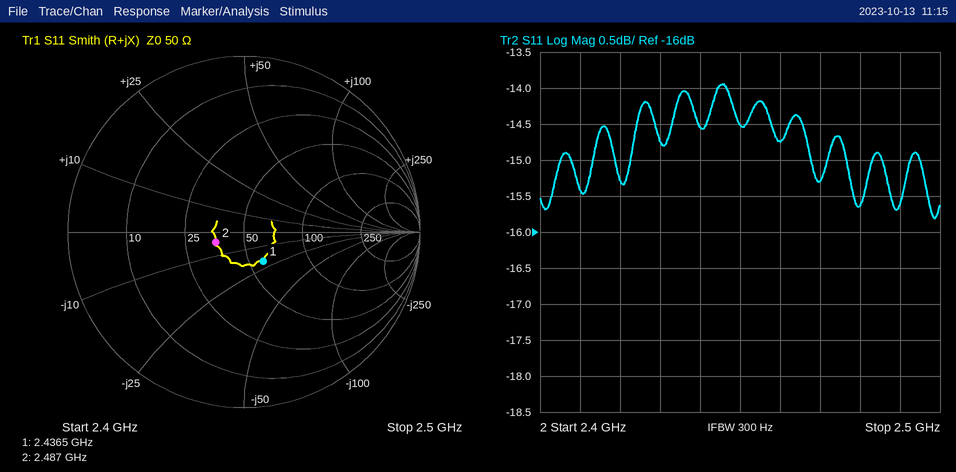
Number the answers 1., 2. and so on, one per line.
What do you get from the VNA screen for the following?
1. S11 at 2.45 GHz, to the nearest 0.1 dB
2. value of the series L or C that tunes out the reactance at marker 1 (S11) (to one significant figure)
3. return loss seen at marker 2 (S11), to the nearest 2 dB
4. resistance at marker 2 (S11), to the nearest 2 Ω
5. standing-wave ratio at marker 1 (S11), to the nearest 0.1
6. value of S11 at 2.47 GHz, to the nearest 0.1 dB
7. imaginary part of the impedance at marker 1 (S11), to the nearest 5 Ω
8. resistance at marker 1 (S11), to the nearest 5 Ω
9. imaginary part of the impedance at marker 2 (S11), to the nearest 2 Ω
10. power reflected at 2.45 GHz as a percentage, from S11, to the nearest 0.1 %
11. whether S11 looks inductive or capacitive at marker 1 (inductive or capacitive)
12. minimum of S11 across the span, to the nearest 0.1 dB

1. -14.5 dB
2. 1 nH
3. 16 dB
4. 36 Ω
5. 1.5
6. -15.3 dB
7. -20 Ω
8. 60 Ω
9. -4 Ω
10. 3.5 %
11. capacitive
12. -15.8 dB
